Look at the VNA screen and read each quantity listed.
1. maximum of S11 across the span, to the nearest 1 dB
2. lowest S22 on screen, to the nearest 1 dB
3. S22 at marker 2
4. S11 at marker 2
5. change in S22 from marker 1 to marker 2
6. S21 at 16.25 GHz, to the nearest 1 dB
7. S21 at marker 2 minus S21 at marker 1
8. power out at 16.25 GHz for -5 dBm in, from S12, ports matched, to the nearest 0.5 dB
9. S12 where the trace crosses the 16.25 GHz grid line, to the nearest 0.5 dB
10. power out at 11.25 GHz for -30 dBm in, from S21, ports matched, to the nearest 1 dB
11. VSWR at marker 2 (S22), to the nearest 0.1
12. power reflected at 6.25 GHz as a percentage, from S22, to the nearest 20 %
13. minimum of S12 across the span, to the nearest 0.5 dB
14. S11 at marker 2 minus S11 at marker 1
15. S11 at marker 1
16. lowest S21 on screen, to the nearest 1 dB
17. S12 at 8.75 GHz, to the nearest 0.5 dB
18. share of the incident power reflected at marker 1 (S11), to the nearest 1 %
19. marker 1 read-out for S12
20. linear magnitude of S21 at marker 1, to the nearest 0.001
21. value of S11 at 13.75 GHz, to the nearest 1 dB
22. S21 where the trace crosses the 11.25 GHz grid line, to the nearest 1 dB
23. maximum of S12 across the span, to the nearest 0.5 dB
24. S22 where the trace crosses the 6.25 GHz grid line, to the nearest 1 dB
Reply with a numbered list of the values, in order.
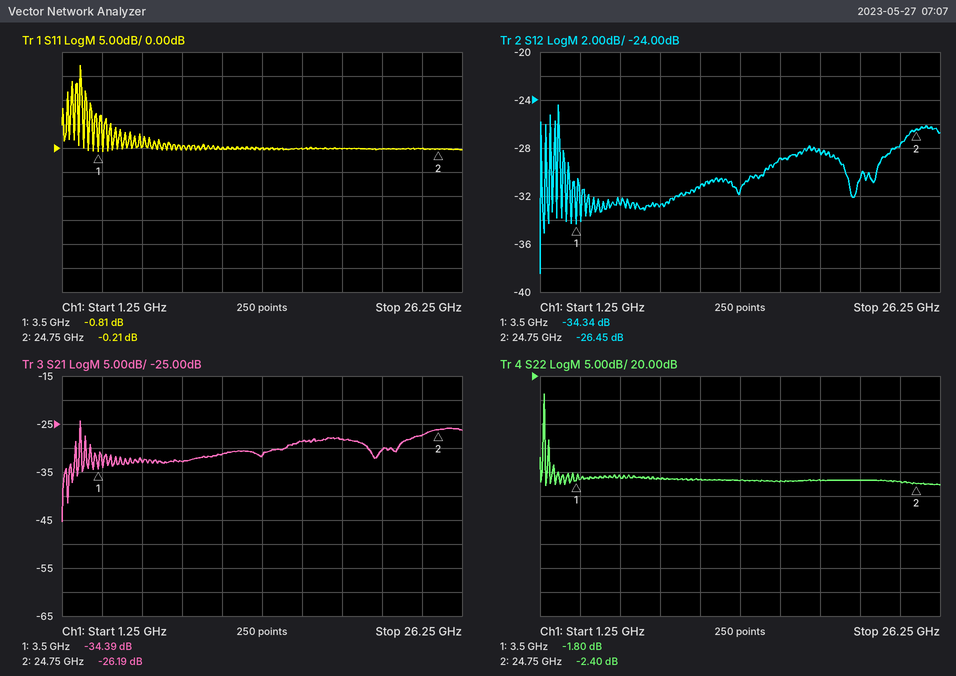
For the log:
1. 17 dB
2. -3 dB
3. -2.40 dB
4. -0.21 dB
5. -0.60 dB
6. -29 dB
7. 8.20 dB
8. -34.0 dBm
9. -29.0 dB
10. -61 dBm
11. 7.3
12. 80 %
13. -38.5 dB
14. 0.60 dB
15. -0.81 dB
16. -45 dB
17. -33.0 dB
18. 83 %
19. -34.34 dB
20. 0.019
21. 0 dB
22. -31 dB
23. -24.5 dB
24. -1 dB
